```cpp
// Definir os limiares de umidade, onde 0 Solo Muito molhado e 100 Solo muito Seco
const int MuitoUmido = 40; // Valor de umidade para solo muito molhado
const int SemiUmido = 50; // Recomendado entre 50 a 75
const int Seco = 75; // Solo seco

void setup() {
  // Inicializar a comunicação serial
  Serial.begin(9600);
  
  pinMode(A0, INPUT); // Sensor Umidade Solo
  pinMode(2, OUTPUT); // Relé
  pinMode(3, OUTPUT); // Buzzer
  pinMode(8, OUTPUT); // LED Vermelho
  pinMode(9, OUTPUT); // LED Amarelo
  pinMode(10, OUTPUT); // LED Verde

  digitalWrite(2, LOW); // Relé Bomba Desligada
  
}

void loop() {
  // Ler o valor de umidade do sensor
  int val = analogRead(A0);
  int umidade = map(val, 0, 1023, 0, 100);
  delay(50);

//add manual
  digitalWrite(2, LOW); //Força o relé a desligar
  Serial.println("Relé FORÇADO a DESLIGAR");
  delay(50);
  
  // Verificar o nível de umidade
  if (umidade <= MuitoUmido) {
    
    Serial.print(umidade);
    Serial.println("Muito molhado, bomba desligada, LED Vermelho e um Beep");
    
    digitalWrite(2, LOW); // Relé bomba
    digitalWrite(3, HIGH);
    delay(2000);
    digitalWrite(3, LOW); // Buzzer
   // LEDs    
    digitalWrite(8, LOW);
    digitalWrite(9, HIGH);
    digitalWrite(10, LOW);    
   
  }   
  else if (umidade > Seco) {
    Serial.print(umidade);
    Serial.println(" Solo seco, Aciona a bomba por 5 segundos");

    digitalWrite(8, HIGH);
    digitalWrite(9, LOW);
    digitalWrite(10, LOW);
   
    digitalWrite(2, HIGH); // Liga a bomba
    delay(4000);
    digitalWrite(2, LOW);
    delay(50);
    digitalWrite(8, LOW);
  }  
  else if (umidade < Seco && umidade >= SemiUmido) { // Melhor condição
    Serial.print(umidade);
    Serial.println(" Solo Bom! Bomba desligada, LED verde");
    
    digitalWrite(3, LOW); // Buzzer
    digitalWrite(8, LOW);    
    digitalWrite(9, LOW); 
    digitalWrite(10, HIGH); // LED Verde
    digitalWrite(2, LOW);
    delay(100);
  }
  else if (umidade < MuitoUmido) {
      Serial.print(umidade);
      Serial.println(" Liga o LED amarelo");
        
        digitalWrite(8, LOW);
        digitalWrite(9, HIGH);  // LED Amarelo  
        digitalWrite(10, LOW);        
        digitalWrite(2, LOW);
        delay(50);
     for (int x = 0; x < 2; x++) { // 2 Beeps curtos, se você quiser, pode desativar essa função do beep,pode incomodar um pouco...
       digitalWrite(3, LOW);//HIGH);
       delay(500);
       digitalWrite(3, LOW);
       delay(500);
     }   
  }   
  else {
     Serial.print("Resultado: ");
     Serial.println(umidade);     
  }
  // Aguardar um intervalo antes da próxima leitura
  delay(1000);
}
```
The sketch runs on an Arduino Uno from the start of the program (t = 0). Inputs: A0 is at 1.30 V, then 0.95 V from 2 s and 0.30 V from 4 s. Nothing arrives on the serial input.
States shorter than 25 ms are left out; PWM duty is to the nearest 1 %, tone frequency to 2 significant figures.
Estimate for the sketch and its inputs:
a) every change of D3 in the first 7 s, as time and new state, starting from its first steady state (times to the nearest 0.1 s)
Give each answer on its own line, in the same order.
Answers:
0 s low; 0.1 s high; 2.1 s low; 3.2 s high; 5.2 s low; 6.3 s high
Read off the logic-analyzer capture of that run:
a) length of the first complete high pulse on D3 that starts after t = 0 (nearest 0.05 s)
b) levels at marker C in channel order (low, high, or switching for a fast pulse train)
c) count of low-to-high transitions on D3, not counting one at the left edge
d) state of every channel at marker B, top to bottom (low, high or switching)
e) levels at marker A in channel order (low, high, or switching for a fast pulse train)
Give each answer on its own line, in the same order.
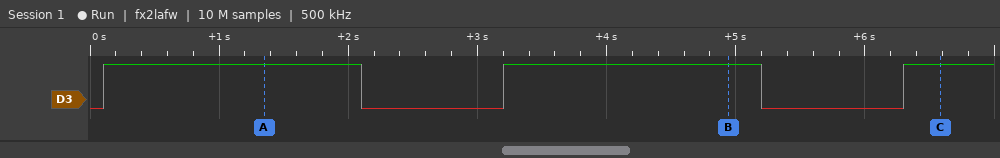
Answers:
2.00 s
D3 high
3
D3 high
D3 high
